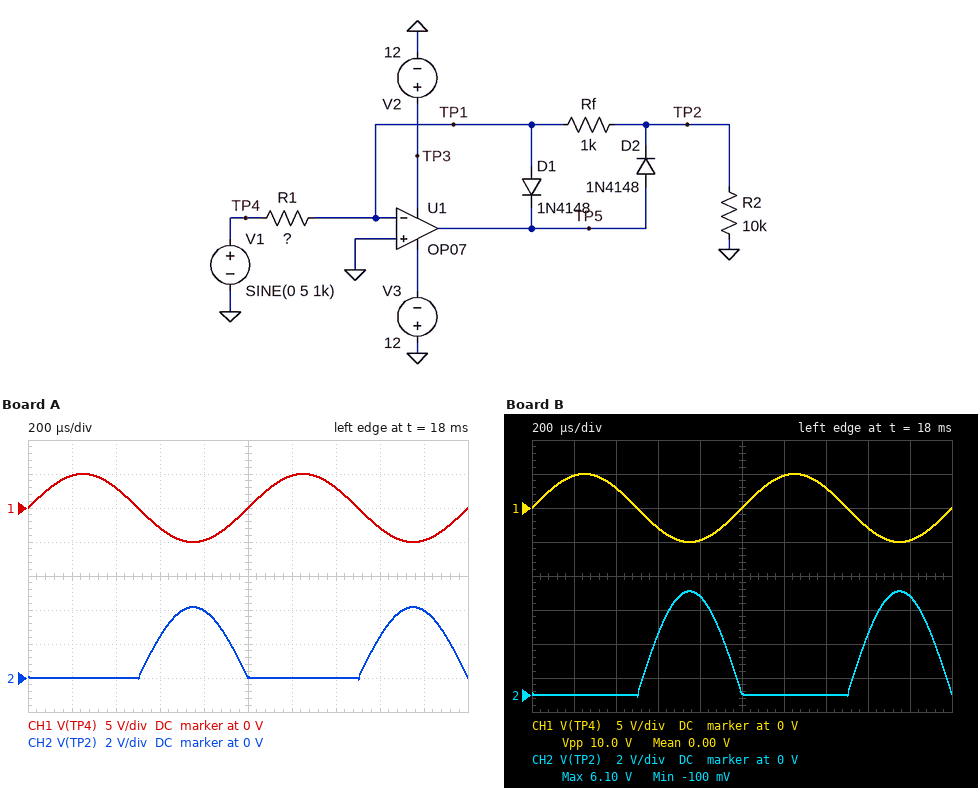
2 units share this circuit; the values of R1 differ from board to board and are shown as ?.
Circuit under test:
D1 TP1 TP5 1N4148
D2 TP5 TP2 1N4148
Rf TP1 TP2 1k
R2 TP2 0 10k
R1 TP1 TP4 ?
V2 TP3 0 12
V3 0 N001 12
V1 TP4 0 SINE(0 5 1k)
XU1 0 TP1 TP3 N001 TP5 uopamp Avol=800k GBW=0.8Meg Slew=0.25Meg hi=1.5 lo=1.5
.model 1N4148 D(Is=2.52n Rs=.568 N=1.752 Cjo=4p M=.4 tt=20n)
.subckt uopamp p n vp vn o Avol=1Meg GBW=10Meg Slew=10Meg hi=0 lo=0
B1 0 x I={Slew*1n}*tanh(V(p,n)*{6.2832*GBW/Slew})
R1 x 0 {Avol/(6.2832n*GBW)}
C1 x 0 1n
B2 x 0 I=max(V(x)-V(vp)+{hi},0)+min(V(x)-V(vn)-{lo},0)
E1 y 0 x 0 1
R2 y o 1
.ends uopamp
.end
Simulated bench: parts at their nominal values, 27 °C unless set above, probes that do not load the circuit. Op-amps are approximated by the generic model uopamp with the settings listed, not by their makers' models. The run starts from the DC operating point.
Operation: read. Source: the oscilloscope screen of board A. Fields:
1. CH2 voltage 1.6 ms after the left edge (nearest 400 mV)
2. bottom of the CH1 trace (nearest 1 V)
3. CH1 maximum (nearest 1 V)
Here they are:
2.4 V
-5 V
5 V
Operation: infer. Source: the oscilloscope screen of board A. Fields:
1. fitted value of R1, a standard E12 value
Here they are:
1.2 kΩ
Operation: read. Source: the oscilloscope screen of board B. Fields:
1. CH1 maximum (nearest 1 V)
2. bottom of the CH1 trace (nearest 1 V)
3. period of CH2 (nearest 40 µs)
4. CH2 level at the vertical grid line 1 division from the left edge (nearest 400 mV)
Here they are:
5 V
-5 V
1.00 ms
0 V
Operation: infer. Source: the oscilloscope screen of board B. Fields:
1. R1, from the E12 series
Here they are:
820 Ω
